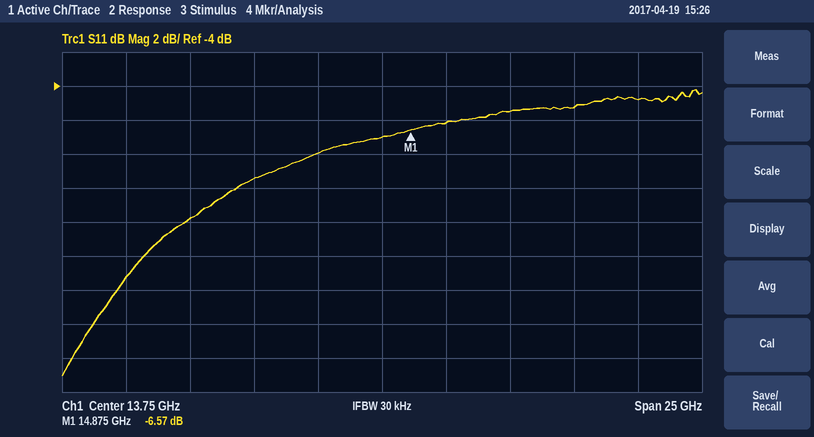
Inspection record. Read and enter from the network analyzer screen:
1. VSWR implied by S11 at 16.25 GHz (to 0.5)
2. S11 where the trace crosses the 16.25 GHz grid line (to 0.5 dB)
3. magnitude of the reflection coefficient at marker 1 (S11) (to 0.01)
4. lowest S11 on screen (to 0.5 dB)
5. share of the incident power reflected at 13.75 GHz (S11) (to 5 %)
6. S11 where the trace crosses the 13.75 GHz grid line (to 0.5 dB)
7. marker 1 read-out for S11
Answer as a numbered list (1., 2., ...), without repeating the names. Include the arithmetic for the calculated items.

1. |Γ| = 10^(-6/20) = 0.5012; VSWR = (1 + 0.5012)/(1 − 0.5012) ≈ 3.0
2. -6.0 dB
3. 10^(-6.57/20) ≈ 0.47
4. -21.0 dB
5. 10^(-7/10) ≈ 20 %
6. -7.0 dB
7. -6.57 dB
